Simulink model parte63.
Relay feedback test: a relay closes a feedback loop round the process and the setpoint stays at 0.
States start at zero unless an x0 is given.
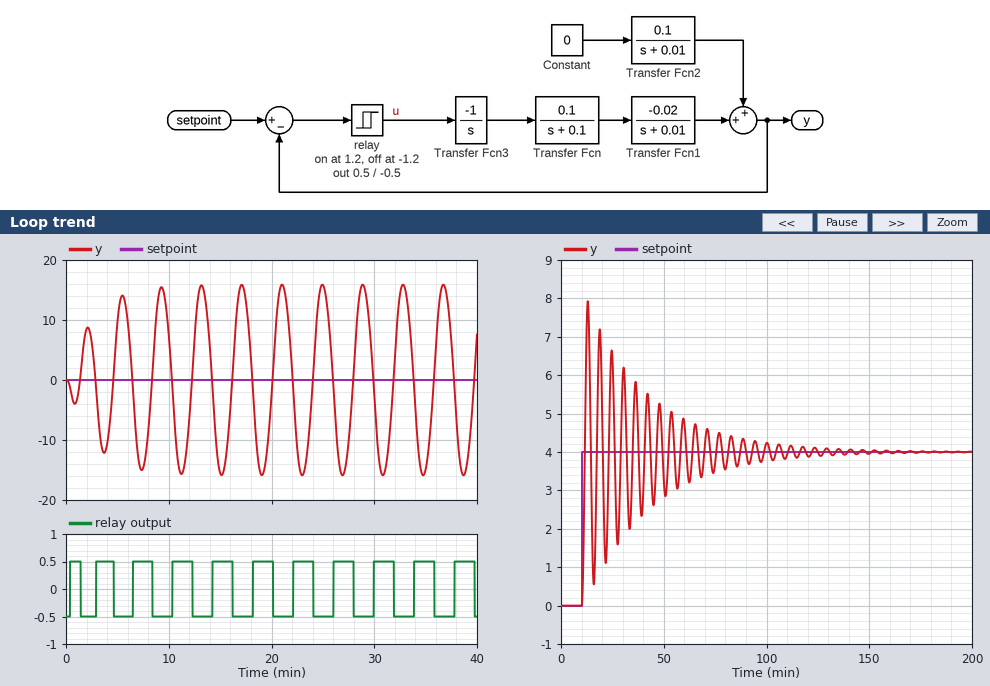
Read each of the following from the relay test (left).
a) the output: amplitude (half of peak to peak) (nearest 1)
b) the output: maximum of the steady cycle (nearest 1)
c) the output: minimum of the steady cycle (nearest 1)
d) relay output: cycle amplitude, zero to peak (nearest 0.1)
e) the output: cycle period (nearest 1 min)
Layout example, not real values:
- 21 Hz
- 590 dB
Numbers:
- 16
- 16
- -16
- 0.5
- 4 min
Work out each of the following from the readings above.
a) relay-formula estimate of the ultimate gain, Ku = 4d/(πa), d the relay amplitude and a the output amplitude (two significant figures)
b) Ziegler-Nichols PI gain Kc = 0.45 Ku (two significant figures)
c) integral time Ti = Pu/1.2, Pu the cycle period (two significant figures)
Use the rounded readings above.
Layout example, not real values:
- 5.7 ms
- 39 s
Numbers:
- 0.040
- 0.018
- 3.3 min
